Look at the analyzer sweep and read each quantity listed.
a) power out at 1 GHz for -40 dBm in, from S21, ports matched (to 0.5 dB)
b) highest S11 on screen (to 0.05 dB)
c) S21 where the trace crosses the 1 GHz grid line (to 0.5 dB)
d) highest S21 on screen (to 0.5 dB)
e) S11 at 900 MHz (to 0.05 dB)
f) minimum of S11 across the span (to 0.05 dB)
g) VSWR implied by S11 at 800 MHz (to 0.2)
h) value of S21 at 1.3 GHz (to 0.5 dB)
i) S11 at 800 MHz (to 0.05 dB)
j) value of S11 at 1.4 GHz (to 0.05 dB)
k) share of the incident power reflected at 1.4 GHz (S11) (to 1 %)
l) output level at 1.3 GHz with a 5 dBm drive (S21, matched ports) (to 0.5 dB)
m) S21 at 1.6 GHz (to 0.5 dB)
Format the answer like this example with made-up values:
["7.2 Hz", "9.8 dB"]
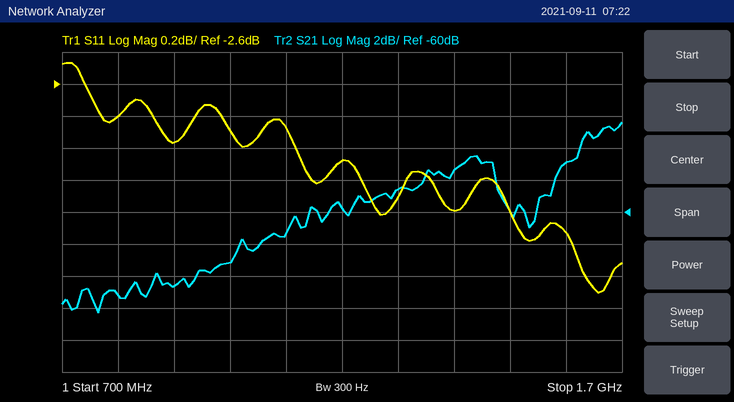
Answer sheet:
["-103.0 dBm", "-2.45 dB", "-63.0 dB", "-54.5 dB", "-2.95 dB", "-3.90 dB", "6.2", "-58.5 dB", "-2.80 dB", "-3.40 dB", "46 %", "-53.5 dBm", "-57.0 dB"]
